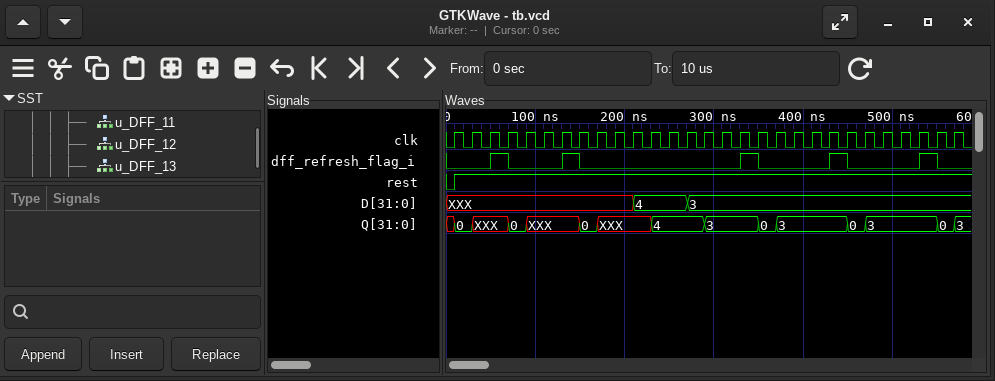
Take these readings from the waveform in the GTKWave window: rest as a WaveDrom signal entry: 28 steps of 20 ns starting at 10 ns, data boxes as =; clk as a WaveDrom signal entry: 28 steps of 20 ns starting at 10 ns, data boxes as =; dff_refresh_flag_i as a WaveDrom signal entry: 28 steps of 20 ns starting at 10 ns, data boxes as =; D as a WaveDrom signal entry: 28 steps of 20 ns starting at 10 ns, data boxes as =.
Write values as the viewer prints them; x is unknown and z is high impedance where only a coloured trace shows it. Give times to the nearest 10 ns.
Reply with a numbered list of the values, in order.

1. {name: 'rest', wave: '1...........................'}
2. {name: 'clk', wave: 'p...........................'}
3. {name: 'dff_refresh_flag_i', wave: '0.10..10........10...10...10'}
4. {name: 'D', wave: 'x.........=..=..............', data: '4 3'}
